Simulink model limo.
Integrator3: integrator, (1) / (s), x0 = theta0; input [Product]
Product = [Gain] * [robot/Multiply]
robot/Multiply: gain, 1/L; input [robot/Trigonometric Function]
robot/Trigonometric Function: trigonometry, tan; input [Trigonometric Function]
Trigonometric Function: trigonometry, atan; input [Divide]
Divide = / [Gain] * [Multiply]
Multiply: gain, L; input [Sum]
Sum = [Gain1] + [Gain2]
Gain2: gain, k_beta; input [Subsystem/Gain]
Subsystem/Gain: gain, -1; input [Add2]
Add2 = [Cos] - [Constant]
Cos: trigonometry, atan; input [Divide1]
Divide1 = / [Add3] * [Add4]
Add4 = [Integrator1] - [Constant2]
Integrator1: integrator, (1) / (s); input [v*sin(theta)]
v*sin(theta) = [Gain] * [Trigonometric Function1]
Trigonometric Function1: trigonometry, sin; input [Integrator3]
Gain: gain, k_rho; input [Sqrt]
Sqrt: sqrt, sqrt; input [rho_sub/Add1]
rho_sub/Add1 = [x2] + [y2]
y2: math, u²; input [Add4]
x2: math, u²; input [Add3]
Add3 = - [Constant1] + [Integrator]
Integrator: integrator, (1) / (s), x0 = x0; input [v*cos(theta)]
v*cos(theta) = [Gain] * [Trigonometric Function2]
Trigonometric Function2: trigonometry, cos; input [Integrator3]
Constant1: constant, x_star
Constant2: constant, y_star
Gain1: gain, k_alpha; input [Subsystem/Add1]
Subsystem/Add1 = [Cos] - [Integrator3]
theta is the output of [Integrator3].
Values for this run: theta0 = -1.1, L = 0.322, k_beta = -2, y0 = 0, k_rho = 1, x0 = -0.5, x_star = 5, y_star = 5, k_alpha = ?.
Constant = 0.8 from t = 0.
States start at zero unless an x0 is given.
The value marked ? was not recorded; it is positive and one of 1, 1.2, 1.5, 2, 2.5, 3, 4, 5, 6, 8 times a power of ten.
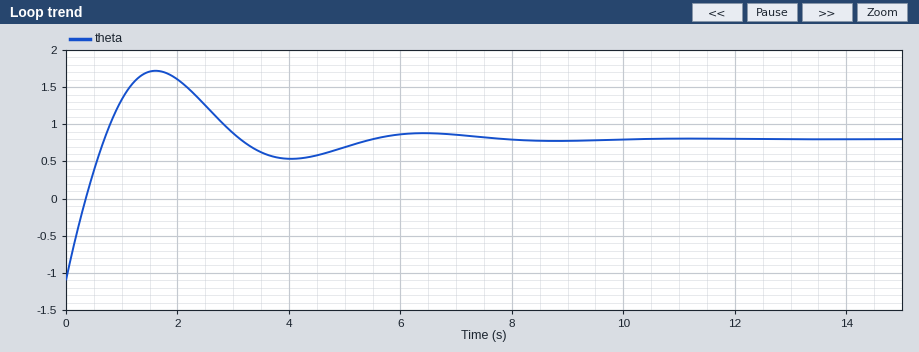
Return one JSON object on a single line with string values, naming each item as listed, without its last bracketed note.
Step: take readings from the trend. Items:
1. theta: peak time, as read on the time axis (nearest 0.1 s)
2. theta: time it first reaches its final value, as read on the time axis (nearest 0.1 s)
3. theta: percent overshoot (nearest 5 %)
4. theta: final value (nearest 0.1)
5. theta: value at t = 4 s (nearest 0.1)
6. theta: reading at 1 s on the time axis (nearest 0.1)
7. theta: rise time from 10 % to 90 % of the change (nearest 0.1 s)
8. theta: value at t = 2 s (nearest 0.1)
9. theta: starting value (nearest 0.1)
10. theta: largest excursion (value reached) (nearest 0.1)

{"theta: peak time, as read on the time axis": "1.6 s", "theta: time it first reaches its final value, as read on the time axis": "0.7 s", "theta: percent overshoot": "50 %", "theta: final value": "0.8", "theta: value at t = 4 s": "0.5", "theta: reading at 1 s on the time axis": "1.3", "theta: rise time from 10 % to 90 % of the change": "0.5 s", "theta: value at t = 2 s": "1.6", "theta: starting value": "-1.1", "theta: largest excursion (value reached)": "1.7"}
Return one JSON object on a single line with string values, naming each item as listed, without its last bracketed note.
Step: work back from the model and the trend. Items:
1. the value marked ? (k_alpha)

{"the value marked ?": "2"}
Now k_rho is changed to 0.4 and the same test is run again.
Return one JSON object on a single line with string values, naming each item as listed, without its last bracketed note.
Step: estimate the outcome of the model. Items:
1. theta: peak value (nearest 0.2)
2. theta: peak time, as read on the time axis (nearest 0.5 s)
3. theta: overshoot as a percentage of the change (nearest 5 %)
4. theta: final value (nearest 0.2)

{"theta: peak value": "1.2", "theta: peak time, as read on the time axis": "2.0 s", "theta: overshoot as a percentage of the change": "20 %", "theta: final value": "0.8"}
